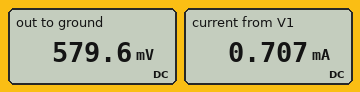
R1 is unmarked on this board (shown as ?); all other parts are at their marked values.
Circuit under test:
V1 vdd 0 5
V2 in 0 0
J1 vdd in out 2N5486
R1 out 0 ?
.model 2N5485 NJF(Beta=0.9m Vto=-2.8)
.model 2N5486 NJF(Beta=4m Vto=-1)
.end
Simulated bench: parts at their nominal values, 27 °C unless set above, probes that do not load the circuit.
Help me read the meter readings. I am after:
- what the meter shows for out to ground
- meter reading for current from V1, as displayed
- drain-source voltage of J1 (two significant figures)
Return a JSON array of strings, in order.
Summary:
["579.6 mV", "0.707 mA", "4.4 V"]
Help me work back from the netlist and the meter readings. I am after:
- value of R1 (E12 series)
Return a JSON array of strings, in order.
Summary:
["820 Ω"]
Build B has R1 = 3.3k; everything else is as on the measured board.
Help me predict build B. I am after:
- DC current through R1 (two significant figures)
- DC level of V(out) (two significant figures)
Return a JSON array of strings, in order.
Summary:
["230 µA", "760 mV"]
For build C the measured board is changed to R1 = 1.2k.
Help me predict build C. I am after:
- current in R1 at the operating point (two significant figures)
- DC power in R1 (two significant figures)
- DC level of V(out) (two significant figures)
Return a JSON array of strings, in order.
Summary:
["530 µA", "340 µW", "640 mV"]
